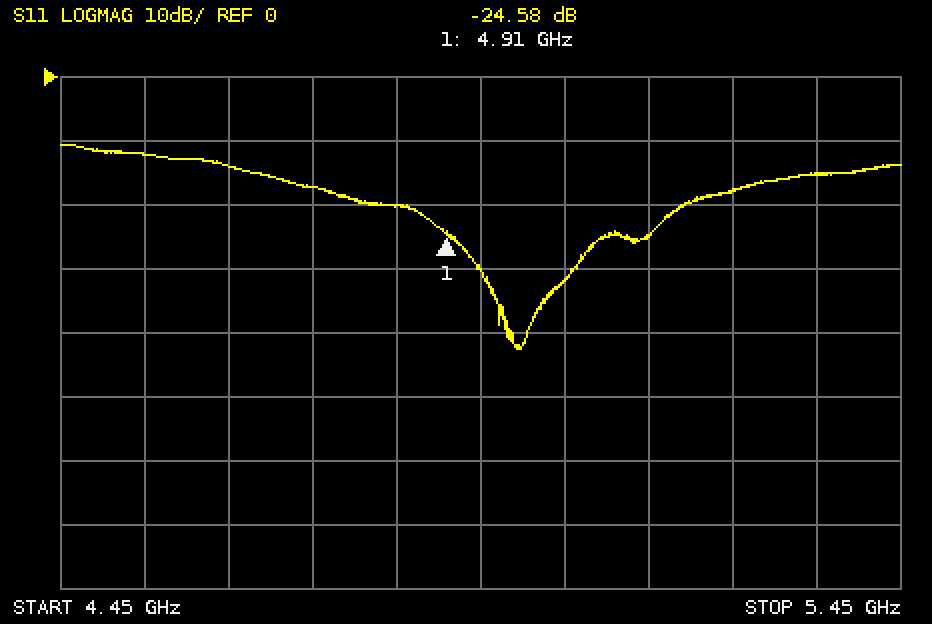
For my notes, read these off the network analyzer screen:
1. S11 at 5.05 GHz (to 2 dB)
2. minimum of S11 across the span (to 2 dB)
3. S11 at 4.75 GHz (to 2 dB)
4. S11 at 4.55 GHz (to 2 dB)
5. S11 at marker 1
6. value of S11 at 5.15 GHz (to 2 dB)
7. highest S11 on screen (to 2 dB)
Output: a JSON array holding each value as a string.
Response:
["-32 dB", "-42 dB", "-18 dB", "-12 dB", "-24.58 dB", "-24 dB", "-10 dB"]
